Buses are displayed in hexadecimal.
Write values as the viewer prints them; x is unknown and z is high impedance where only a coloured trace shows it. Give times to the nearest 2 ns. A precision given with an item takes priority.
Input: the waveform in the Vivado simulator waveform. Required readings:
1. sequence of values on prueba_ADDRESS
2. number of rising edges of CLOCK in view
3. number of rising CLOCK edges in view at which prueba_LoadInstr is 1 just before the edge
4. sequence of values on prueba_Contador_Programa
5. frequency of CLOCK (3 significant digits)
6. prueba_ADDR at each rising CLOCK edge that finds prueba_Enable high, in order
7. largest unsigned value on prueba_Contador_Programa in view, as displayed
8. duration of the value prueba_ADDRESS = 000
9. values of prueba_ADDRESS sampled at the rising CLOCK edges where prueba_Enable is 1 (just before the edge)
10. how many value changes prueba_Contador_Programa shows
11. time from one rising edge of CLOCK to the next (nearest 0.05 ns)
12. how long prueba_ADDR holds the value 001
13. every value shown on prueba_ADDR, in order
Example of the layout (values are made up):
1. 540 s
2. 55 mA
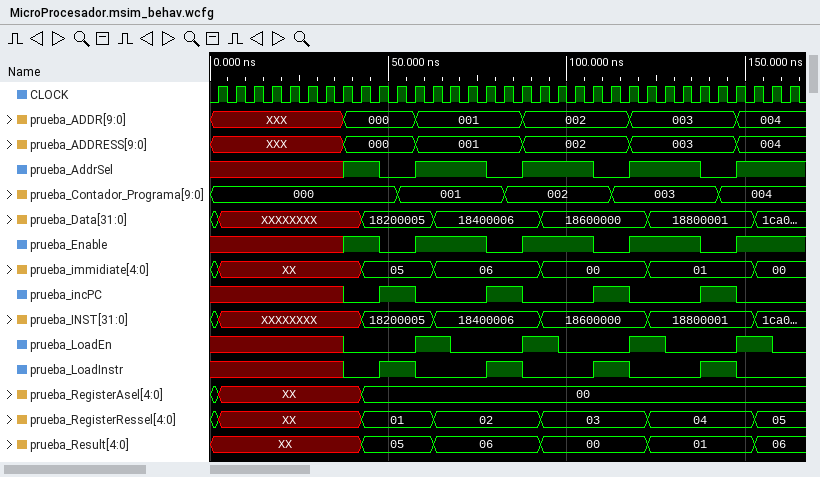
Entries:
1. XXX, 000, 001, 002, 003, 004
2. 33
3. 8
4. 000, 001, 002, 003, 004
5. 200 MHz
6. 000, 000, 001, 001, 001, 001, 002, 002, 002, 002, 003, 003, 003, 003, 004, 004, 004
7. 004
8. 20 ns
9. 000, 000, 001, 001, 001, 001, 002, 002, 002, 002, 003, 003, 003, 003, 004, 004, 004
10. 4
11. 5 ns
12. 30 ns
13. XXX, 000, 001, 002, 003, 004
